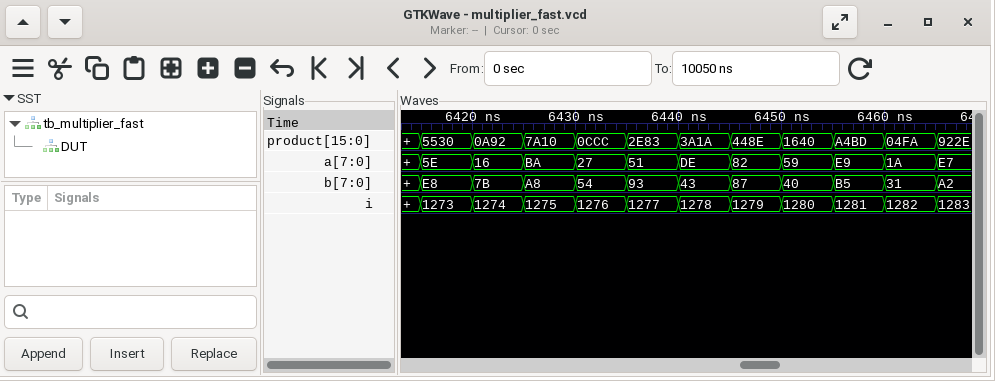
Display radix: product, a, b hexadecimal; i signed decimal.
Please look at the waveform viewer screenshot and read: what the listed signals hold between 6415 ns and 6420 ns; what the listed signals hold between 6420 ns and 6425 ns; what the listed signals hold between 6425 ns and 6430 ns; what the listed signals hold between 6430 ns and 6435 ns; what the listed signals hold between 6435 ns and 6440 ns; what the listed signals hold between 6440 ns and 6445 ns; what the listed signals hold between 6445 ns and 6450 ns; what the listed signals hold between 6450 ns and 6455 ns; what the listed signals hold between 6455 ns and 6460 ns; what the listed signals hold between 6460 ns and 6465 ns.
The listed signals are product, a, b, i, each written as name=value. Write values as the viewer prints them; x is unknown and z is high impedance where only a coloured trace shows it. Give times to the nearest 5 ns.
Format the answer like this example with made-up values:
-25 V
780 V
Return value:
product=5530, a=5E, b=E8, i=1273
product=0A92, a=16, b=7B, i=1274
product=7A10, a=BA, b=A8, i=1275
product=0CCC, a=27, b=54, i=1276
product=2E83, a=51, b=93, i=1277
product=3A1A, a=DE, b=43, i=1278
product=448E, a=82, b=87, i=1279
product=1640, a=59, b=40, i=1280
product=A4BD, a=E9, b=B5, i=1281
product=04FA, a=1A, b=31, i=1282
